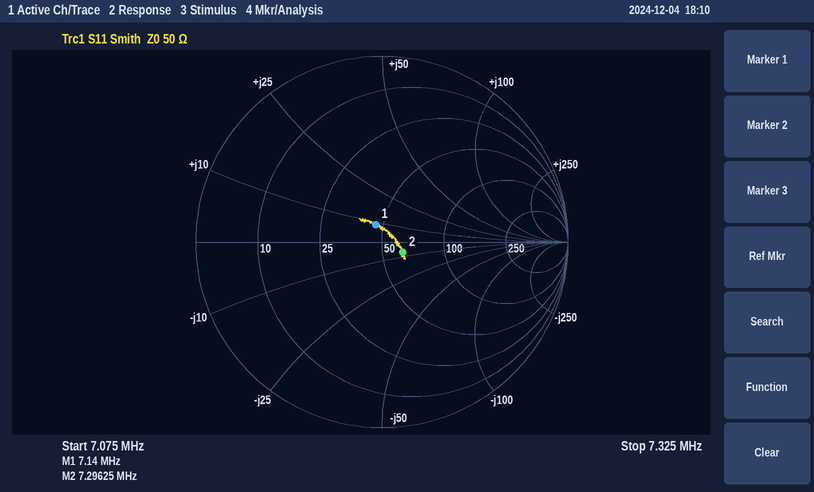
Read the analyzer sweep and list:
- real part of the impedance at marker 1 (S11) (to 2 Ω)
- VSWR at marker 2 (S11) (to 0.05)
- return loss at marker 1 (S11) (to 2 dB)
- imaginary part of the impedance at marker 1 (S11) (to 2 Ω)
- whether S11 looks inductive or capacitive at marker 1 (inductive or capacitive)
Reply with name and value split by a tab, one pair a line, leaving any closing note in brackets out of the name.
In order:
real part of the impedance at marker 1 (S11)	46 Ω
VSWR at marker 2 (S11)	1.30
return loss at marker 1 (S11)	20 dB
imaginary part of the impedance at marker 1 (S11)	+8 Ω
whether S11 looks inductive or capacitive at marker 1	inductive
